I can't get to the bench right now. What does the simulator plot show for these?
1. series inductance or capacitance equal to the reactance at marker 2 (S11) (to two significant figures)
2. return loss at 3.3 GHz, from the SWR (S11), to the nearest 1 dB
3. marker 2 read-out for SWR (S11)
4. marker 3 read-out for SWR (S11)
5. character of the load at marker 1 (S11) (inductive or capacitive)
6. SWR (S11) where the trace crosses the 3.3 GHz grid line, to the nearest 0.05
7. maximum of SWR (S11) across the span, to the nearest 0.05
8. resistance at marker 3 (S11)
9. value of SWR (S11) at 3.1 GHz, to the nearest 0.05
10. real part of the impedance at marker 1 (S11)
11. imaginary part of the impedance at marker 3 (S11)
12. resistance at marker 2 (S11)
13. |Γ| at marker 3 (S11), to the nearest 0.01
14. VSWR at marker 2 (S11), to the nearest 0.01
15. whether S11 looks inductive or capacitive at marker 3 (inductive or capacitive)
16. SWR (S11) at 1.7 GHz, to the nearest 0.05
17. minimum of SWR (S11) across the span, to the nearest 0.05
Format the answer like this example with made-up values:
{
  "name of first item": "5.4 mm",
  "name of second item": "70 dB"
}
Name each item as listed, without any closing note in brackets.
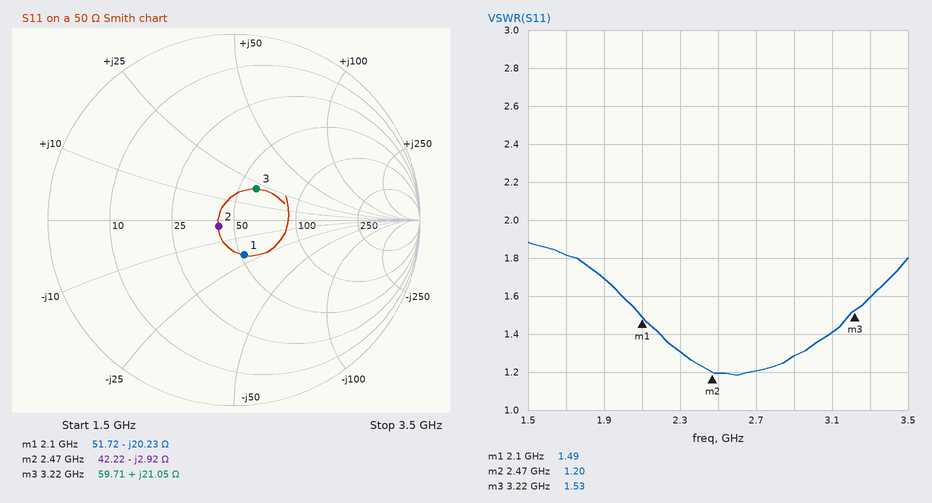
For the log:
{
  "series inductance or capacitance equal to the reactance at marker 2 (S11)": "22 pF",
  "return loss at 3.3 GHz, from the SWR (S11), to the nearest 1 dB": "13 dB",
  "marker 2 read-out for SWR": "1.20",
  "marker 3 read-out for SWR": "1.53",
  "character of the load at marker 1 (S11)": "capacitive",
  "SWR (S11) where the trace crosses the 3.3 GHz grid line, to the nearest 0.05": "1.60",
  "maximum of SWR (S11) across the span, to the nearest 0.05": "1.90",
  "resistance at marker 3": "59.71 Ω",
  "value of SWR (S11) at 3.1 GHz, to the nearest 0.05": "1.40",
  "real part of the impedance at marker 1": "51.72 Ω",
  "imaginary part of the impedance at marker 3": "+21.05 Ω",
  "resistance at marker 2": "42.22 Ω",
  "|Γ| at marker 3 (S11), to the nearest 0.01": "0.21",
  "VSWR at marker 2 (S11), to the nearest 0.01": "1.20",
  "whether S11 looks inductive or capacitive at marker 3": "inductive",
  "SWR (S11) at 1.7 GHz, to the nearest 0.05": "1.80",
  "minimum of SWR (S11) across the span, to the nearest 0.05": "1.20"
}
